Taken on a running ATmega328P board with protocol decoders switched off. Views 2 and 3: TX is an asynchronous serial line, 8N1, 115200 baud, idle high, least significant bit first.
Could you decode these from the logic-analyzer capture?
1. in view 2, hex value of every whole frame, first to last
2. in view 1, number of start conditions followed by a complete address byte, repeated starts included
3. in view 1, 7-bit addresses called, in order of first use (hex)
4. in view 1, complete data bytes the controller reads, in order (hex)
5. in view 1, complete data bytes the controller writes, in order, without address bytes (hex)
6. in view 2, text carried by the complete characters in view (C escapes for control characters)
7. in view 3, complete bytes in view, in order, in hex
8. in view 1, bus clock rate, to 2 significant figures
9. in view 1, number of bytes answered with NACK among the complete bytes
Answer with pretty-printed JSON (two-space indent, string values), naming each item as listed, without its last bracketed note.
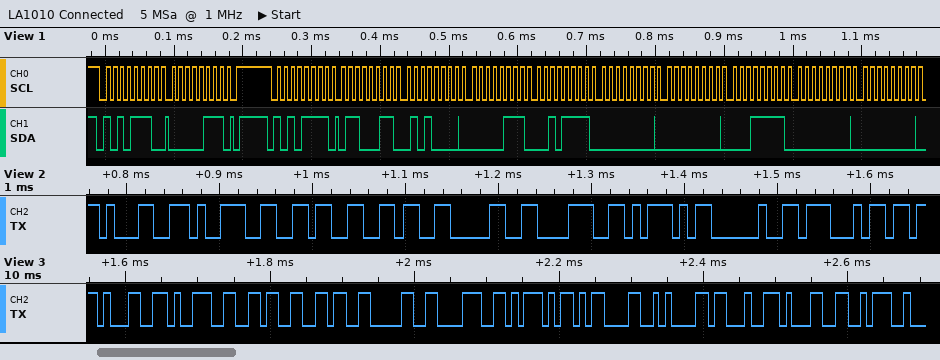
{
  "in view 2, hex value of every whole frame, first to last": "31 39 36 36 30 38 5D 20 47",
  "in view 1, number of start conditions followed by a complete address byte, repeated starts included": "2",
  "in view 1, 7-bit addresses called, in order of first use": "0x57",
  "in view 1, complete data bytes the controller reads, in order": "63 50 07 2F 00 00 1F 00 00",
  "in view 1, complete data bytes the controller writes, in order, without address bytes": "07",
  "in view 2, text carried by the complete characters in view": "\"196608] G\"",
  "in view 3, complete bytes in view, in order, in hex": "31 39 36 36 30 38 5D 0D 0A 23 31 3A",
  "in view 1, bus clock rate, to 2 significant figures": "100 kHz",
  "in view 1, number of bytes answered with NACK among the complete bytes": "0"
}
